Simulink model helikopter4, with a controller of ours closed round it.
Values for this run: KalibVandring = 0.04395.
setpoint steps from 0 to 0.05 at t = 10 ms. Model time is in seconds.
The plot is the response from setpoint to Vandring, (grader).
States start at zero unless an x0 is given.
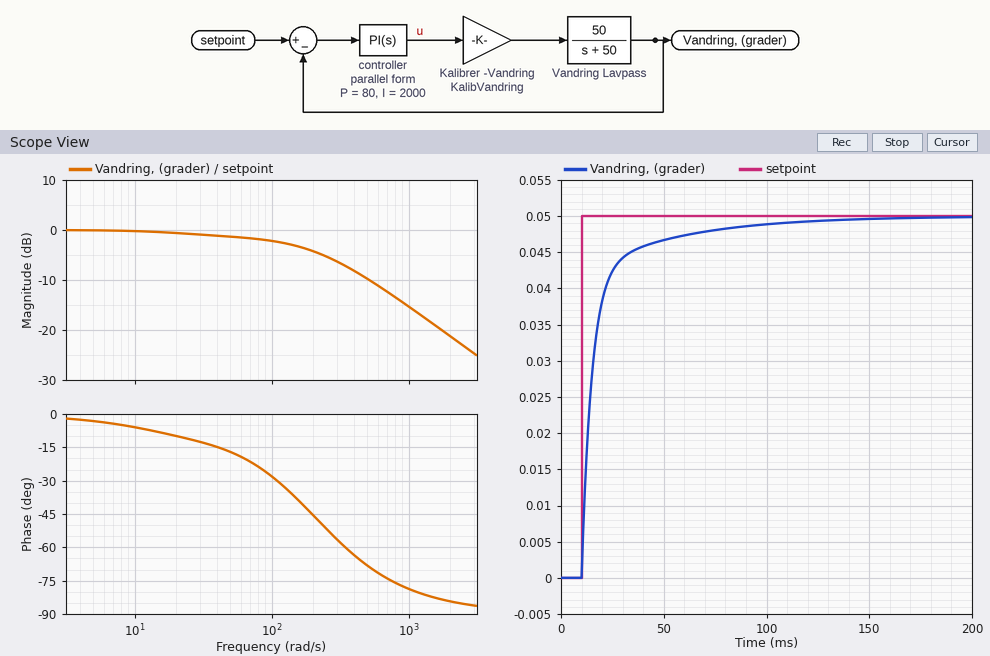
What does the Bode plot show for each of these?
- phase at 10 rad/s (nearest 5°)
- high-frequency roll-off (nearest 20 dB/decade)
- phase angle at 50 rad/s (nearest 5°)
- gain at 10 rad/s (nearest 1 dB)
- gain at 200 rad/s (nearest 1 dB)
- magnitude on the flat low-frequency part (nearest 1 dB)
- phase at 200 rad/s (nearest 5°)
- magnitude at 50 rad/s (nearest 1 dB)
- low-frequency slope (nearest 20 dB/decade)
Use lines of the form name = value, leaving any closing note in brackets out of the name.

phase at 10 rad/s = -5°
high-frequency roll-off = -20 dB/decade
phase angle at 50 rad/s = -15°
gain at 10 rad/s = 0 dB
gain at 200 rad/s = -4 dB
magnitude on the flat low-frequency part = 0 dB
phase at 200 rad/s = -45°
magnitude at 50 rad/s = -1 dB
low-frequency slope = 0 dB/decade
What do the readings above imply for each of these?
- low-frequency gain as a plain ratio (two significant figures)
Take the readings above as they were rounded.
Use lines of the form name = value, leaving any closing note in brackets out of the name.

low-frequency gain as a plain ratio = 1.0
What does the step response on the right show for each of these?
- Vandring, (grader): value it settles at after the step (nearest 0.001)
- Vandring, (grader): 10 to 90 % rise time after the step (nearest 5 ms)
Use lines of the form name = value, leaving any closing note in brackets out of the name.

Vandring, (grader): value it settles at after the step = 0.050
Vandring, (grader): 10 to 90 % rise time after the step = 25 ms
